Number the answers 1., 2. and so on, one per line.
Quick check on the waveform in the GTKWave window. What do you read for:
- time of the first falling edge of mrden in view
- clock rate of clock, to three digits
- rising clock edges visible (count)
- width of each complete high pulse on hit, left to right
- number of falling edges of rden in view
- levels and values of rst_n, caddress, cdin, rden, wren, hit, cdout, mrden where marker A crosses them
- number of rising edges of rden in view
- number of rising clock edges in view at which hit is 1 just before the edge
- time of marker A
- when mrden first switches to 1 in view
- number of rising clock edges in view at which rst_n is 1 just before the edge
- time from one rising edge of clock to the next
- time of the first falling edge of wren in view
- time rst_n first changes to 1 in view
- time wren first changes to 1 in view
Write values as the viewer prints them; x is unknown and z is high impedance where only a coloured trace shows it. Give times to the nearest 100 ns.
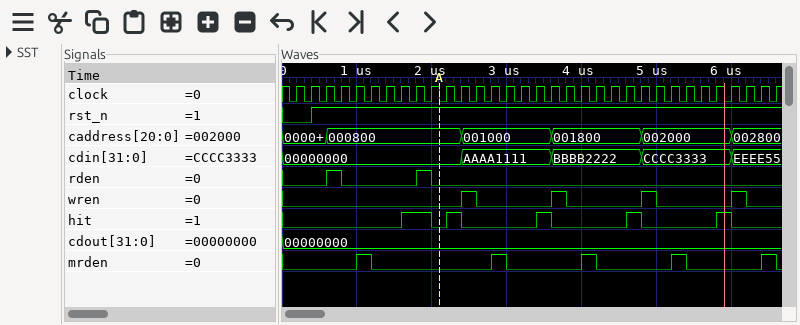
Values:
1. 1200 ns
2. 5.00 MHz
3. 33
4. 400 ns, 200 ns, 200 ns, 200 ns, 200 ns
5. 2
6. rst_n=1, caddress=000800, cdin=00000000, rden=0, wren=0, hit=0, cdout=00000000, mrden=0
7. 2
8. 6
9. 2100 ns
10. 1000 ns
11. 31
12. 200 ns
13. 2600 ns
14. 400 ns
15. 2400 ns
